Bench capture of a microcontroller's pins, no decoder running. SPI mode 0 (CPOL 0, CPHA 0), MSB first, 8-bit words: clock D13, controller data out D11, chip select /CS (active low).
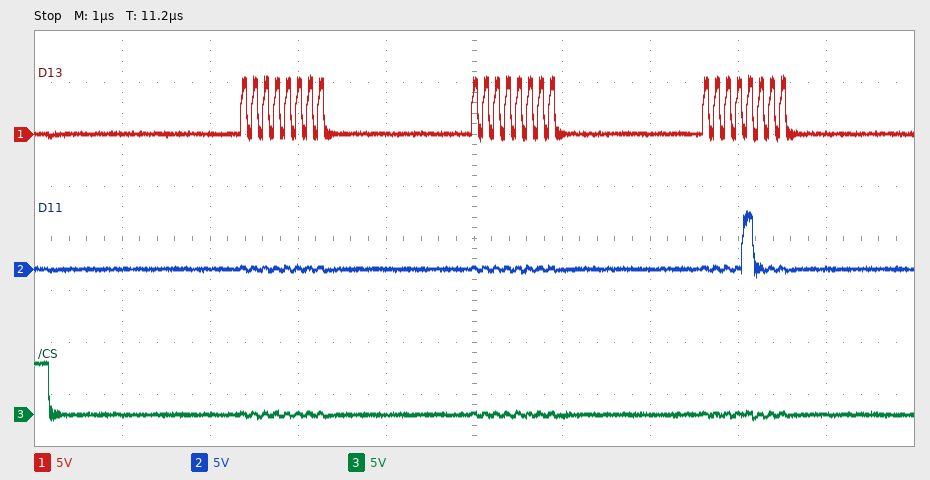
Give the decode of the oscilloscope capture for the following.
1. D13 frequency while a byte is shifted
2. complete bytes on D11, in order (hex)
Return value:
8 MHz
00 00 08
